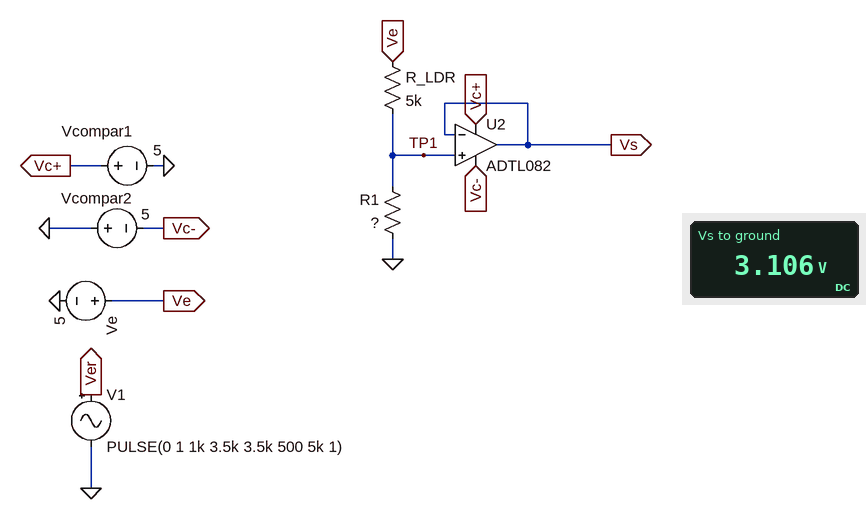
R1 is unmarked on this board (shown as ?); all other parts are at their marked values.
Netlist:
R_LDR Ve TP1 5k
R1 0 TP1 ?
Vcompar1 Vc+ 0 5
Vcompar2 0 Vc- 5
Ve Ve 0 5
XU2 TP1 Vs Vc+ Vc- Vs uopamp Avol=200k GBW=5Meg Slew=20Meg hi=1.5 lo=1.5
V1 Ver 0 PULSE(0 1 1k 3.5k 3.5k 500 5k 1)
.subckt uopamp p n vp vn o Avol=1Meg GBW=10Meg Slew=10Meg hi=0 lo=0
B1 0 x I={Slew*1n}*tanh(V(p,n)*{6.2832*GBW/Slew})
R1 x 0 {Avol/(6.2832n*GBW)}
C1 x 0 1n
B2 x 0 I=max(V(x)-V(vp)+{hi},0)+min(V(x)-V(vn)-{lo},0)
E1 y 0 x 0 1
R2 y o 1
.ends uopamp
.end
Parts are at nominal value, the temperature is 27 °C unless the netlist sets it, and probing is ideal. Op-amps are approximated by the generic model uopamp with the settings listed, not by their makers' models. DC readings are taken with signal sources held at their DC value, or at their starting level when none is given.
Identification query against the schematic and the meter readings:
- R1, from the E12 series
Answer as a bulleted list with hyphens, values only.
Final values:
- 8.2 kΩ
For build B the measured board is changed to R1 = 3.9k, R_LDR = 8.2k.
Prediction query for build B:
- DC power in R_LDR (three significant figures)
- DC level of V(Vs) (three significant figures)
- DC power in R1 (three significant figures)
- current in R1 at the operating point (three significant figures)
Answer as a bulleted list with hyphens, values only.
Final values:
- 1.40 mW
- 1.61 V
- 666 µW
- 413 µA
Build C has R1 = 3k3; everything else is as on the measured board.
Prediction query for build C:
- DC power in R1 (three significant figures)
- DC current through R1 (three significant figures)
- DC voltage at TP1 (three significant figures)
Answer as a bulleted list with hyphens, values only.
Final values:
- 1.20 mW
- 602 µA
- 1.99 V
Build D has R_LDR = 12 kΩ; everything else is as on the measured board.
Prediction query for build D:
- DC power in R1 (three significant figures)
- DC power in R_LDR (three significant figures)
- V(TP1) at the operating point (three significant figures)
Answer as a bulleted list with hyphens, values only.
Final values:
- 502 µW
- 735 µW
- 2.03 V
